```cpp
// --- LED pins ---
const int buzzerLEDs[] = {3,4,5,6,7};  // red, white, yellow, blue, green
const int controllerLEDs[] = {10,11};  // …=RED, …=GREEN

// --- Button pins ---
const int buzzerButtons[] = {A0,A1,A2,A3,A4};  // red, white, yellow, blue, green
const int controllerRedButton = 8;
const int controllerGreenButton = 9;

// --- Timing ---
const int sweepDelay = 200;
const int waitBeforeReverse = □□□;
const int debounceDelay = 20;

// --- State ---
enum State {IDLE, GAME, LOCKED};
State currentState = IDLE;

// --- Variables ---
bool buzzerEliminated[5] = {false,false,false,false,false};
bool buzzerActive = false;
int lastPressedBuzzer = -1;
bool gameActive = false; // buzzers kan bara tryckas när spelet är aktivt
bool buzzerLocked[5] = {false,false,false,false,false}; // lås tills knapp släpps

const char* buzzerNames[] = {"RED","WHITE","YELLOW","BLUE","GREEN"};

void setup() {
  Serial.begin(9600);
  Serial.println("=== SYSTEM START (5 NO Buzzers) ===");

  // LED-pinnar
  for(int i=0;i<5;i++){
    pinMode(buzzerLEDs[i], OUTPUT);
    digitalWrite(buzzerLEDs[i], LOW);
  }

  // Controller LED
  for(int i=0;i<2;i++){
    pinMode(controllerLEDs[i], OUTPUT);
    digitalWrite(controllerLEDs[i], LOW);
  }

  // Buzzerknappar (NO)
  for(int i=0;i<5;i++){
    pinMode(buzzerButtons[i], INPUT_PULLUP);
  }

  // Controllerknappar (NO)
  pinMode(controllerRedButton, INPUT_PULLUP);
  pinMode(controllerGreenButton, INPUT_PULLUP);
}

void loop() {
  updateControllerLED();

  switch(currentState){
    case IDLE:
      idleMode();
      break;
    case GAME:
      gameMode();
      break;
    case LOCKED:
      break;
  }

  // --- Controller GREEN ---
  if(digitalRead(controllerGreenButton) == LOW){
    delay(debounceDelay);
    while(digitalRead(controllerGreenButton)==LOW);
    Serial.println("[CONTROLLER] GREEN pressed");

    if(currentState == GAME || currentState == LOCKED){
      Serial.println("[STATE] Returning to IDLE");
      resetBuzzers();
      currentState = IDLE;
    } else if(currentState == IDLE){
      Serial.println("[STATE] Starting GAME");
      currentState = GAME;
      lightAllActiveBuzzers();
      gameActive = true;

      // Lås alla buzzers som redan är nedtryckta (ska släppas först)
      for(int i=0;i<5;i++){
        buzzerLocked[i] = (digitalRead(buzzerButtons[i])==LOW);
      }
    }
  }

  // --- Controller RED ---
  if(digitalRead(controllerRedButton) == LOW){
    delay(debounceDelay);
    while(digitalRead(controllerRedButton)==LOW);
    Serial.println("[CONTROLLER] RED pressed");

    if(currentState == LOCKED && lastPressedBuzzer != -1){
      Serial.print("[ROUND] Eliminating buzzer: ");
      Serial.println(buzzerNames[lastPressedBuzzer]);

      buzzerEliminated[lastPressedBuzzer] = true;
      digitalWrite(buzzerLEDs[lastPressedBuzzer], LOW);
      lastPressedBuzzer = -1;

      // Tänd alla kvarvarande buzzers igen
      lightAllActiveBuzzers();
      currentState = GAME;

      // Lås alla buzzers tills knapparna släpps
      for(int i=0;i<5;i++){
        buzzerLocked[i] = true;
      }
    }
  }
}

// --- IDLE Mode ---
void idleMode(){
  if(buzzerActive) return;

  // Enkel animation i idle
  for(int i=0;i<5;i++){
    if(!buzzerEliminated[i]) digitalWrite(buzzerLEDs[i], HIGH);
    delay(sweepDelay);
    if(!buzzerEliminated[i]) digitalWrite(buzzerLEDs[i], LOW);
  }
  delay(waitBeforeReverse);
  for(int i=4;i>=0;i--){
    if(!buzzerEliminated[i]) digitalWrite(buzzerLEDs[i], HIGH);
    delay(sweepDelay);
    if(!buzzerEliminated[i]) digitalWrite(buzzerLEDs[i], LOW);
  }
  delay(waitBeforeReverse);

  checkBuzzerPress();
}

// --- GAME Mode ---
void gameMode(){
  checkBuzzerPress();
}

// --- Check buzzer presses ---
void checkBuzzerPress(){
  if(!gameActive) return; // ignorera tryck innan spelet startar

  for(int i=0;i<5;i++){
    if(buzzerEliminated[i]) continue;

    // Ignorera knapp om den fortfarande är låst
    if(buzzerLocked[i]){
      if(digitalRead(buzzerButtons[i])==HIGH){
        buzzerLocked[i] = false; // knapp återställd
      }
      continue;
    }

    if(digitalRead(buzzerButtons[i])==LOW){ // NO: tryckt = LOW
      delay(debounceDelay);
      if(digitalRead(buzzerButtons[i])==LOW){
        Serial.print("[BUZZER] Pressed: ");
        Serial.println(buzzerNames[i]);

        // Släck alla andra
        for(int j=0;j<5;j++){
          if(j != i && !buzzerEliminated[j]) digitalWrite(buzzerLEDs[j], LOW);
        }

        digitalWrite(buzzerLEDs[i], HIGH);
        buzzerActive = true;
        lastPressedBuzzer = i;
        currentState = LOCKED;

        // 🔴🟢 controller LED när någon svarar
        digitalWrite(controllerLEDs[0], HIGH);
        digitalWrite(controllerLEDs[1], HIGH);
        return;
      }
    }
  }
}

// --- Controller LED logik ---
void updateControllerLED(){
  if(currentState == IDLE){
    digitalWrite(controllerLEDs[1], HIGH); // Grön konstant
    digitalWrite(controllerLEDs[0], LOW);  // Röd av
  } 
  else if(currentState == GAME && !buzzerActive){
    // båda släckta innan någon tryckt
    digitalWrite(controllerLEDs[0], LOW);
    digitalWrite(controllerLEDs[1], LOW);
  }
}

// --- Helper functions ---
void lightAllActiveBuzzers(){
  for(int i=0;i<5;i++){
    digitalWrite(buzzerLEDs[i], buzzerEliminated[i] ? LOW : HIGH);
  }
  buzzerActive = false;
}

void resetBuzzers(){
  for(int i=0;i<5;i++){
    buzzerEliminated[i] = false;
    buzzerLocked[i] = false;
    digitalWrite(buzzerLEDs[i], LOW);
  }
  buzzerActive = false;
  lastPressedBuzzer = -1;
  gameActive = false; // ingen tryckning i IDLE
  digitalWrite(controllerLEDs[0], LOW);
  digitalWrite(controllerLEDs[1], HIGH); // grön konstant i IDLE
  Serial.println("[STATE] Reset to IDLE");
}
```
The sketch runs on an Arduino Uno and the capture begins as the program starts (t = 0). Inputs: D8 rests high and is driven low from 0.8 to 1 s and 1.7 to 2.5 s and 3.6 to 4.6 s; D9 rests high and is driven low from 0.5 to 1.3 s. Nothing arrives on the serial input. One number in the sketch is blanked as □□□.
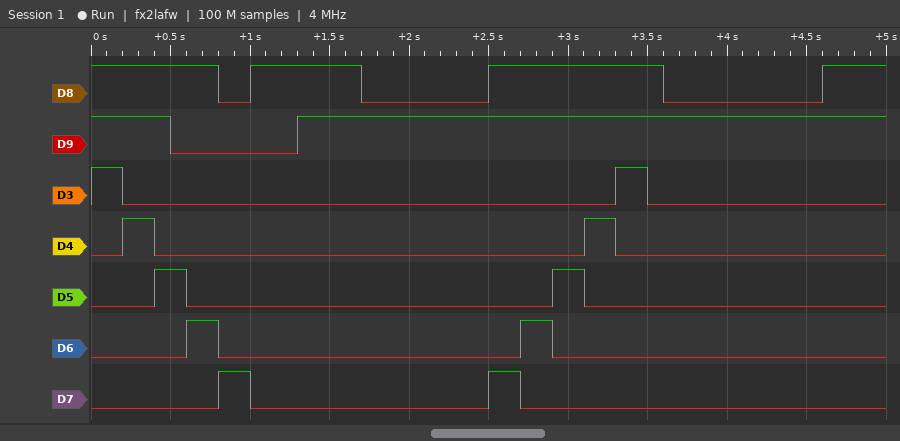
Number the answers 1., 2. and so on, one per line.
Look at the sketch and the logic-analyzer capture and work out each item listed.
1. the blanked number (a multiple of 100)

1. 1500
